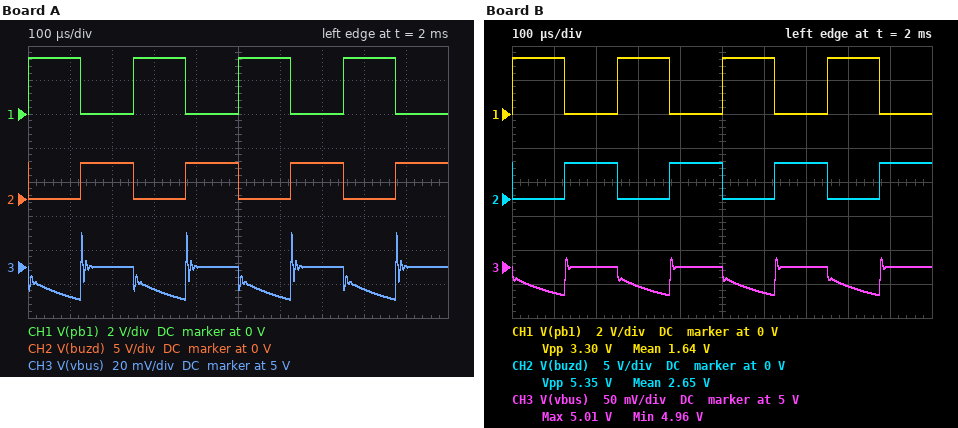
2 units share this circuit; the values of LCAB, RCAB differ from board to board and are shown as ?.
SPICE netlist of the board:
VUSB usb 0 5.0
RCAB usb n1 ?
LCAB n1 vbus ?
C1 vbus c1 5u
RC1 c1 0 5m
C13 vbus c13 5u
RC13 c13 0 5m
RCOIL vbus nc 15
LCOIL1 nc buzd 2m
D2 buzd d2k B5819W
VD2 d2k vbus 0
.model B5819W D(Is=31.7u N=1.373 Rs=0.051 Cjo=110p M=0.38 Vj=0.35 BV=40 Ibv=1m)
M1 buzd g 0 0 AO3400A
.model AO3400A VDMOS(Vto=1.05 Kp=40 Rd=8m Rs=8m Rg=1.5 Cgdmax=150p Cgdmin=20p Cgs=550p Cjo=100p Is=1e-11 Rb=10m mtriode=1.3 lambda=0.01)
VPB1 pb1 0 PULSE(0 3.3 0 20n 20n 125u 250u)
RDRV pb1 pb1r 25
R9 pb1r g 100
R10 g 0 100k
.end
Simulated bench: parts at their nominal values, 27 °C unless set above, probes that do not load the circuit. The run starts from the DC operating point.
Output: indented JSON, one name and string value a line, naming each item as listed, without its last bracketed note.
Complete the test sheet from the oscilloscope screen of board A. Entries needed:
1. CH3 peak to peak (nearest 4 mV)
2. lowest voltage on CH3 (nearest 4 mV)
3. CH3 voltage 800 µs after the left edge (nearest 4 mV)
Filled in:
{
  "CH3 peak to peak": "40 mV",
  "lowest voltage on CH3": "4.980 V",
  "CH3 voltage 800 µs after the left edge": "4.988 V"
}
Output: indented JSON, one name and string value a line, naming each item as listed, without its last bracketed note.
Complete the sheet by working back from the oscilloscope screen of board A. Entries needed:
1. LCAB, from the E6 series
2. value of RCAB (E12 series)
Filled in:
{
  "LCAB, from the E6 series": "220 nH",
  "value of RCAB": "0.082 Ω"
}
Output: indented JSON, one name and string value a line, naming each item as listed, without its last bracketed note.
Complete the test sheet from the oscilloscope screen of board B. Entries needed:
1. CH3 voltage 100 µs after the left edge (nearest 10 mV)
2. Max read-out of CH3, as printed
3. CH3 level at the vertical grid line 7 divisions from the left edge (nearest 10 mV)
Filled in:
{
  "CH3 voltage 100 µs after the left edge": "4.96 V",
  "Max read-out of CH3, as printed": "5.01 V",
  "CH3 level at the vertical grid line 7 divisions from the left edge": "5.00 V"
}
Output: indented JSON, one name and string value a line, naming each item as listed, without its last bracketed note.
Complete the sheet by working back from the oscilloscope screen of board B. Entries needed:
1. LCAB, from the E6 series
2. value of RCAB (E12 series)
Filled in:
{
  "LCAB, from the E6 series": "330 nH",
  "value of RCAB": "0.18 Ω"
}
